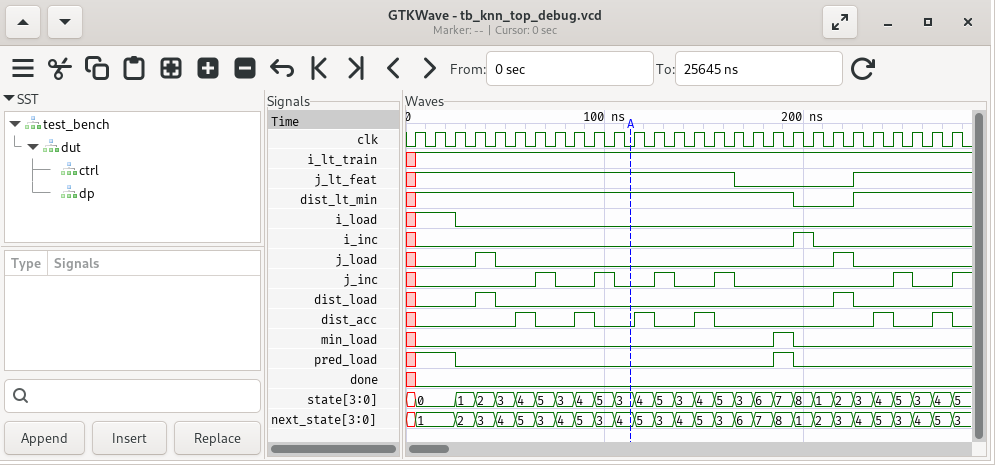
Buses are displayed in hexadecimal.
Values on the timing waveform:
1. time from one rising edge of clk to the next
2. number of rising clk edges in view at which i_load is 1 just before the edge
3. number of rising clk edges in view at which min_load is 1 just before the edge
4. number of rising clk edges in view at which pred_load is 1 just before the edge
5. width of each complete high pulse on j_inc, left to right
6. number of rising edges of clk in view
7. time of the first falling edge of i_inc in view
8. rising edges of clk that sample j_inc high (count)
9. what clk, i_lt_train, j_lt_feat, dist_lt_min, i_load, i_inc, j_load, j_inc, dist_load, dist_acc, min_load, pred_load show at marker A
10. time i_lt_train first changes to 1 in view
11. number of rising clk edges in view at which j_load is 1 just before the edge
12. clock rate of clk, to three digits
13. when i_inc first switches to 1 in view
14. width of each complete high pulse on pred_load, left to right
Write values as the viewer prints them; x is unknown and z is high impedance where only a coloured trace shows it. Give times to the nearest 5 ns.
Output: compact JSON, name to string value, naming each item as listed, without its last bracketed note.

{"time from one rising edge of clk to the next": "10 ns", "number of rising clk edges in view at which i_load is 1 just before the edge": "2", "number of rising clk edges in view at which min_load is 1 just before the edge": "1", "number of rising clk edges in view at which pred_load is 1 just before the edge": "3", "width of each complete high pulse on j_inc, left to right": "10 ns, 10 ns, 10 ns, 10 ns, 10 ns", "number of rising edges of clk in view": "28", "time of the first falling edge of i_inc in view": "205 ns", "rising edges of clk that sample j_inc high": "5", "what clk, i_lt_train, j_lt_feat, dist_lt_min, i_load, i_inc, j_load, j_inc, dist_load, dist_acc, min_load, pred_load show at marker A": "clk=0, i_lt_train=1, j_lt_feat=1, dist_lt_min=1, i_load=0, i_inc=0, j_load=0, j_inc=0, dist_load=0, dist_acc=0, min_load=0, pred_load=0", "time i_lt_train first changes to 1 in view": "5 ns", "number of rising clk edges in view at which j_load is 1 just before the edge": "2", "clock rate of clk, to three digits": "100 MHz", "when i_inc first switches to 1 in view": "195 ns", "width of each complete high pulse on pred_load, left to right": "10 ns"}
